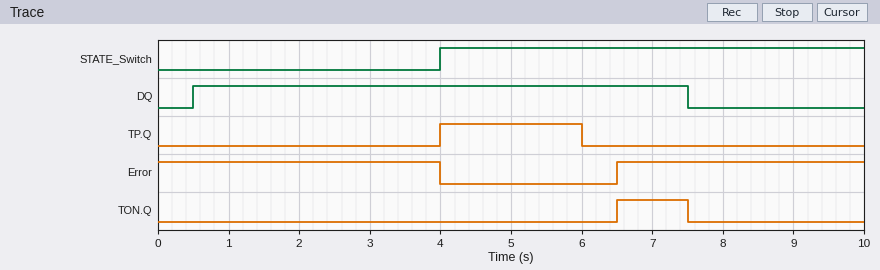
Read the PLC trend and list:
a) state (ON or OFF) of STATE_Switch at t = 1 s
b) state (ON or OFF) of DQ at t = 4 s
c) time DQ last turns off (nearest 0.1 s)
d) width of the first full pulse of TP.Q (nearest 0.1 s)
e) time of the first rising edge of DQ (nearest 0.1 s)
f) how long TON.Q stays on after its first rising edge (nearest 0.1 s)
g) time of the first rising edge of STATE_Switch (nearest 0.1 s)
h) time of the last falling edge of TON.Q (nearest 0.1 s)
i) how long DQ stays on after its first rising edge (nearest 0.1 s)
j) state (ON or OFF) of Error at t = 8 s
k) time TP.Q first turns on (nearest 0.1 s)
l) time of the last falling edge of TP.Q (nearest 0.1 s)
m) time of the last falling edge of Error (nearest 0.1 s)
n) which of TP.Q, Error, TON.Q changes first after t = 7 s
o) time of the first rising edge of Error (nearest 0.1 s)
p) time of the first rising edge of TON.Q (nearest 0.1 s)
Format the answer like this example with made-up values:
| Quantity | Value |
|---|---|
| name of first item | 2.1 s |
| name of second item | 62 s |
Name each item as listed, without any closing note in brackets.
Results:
| Quantity | Value |
|---|---|
| state (ON or OFF) of STATE_Switch at t = 1 s | OFF |
| state (ON or OFF) of DQ at t = 4 s | ON |
| time DQ last turns off | 7.5 s |
| width of the first full pulse of TP.Q | 2.0 s |
| time of the first rising edge of DQ | 0.5 s |
| how long TON.Q stays on after its first rising edge | 1.0 s |
| time of the first rising edge of STATE_Switch | 4.0 s |
| time of the last falling edge of TON.Q | 7.5 s |
| how long DQ stays on after its first rising edge | 7.0 s |
| state (ON or OFF) of Error at t = 8 s | ON |
| time TP.Q first turns on | 4.0 s |
| time of the last falling edge of TP.Q | 6.0 s |
| time of the last falling edge of Error | 4.0 s |
| which of TP.Q, Error, TON.Q changes first after t = 7 s | TON.Q |
| time of the first rising edge of Error | 6.5 s |
| time of the first rising edge of TON.Q | 6.5 s |
